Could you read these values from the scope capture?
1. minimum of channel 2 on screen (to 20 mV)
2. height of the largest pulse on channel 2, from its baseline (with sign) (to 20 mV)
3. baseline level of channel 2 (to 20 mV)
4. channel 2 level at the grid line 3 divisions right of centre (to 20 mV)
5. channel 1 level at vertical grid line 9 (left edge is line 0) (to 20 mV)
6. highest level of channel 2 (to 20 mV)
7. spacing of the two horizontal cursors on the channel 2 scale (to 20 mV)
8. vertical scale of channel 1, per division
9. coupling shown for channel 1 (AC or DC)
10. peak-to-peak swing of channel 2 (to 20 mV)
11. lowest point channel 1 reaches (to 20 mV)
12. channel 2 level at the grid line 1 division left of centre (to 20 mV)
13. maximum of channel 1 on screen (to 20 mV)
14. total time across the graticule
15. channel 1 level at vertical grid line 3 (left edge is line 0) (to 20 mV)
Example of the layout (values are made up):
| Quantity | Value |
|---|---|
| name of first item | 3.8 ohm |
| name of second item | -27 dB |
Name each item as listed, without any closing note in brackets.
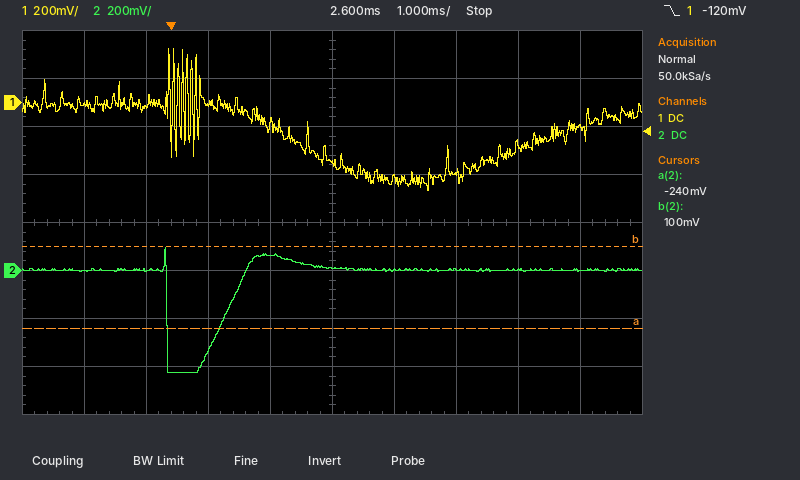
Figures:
| Quantity | Value |
|---|---|
| minimum of channel 2 on screen | -420 mV |
| height of the largest pulse on channel 2, from its baseline (with sign) | -420 mV |
| baseline level of channel 2 | 0 mV |
| channel 2 level at the grid line 3 divisions right of centre | 0 mV |
| channel 1 level at vertical grid line 9 (left edge is line 0) | -100 mV |
| highest level of channel 2 | 100 mV |
| spacing of the two horizontal cursors on the channel 2 scale | 340 mV |
| vertical scale of channel 1, per division | 200 mV |
| coupling shown for channel 1 | DC |
| peak-to-peak swing of channel 2 | 520 mV |
| lowest point channel 1 reaches | -360 mV |
| channel 2 level at the grid line 1 division left of centre | 60 mV |
| maximum of channel 1 on screen | 220 mV |
| total time across the graticule | 10 ms |
| channel 1 level at vertical grid line 3 (left edge is line 0) | 0 mV |
